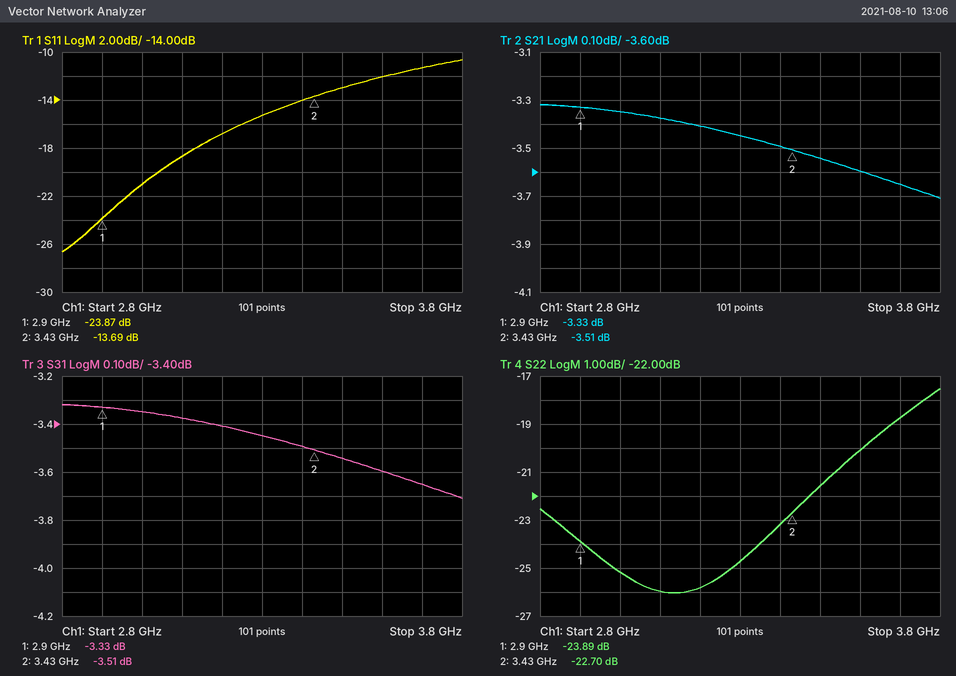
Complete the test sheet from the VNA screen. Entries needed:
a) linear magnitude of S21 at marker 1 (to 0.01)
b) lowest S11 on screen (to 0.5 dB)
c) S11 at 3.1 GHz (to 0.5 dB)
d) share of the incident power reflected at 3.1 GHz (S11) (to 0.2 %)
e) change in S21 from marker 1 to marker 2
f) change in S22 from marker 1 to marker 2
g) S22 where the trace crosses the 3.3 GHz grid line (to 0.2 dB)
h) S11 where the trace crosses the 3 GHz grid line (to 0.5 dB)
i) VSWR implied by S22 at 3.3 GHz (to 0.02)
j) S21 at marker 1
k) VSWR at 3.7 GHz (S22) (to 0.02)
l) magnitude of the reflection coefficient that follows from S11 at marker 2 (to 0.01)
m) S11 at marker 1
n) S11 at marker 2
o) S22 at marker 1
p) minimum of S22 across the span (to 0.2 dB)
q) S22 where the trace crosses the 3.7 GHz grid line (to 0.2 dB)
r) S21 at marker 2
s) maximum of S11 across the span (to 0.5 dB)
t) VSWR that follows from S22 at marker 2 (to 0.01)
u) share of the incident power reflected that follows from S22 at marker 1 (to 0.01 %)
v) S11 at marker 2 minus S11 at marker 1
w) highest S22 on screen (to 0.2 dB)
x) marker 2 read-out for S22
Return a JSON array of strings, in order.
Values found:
["0.68", "-26.5 dB", "-18.5 dB", "1.4 %", "-0.18 dB", "1.19 dB", "-24.8 dB", "-21.0 dB", "1.12", "-3.33 dB", "1.26", "0.21", "-23.87 dB", "-13.69 dB", "-23.89 dB", "-26.0 dB", "-18.8 dB", "-3.51 dB", "-10.5 dB", "1.16", "0.41 %", "10.18 dB", "-17.6 dB", "-22.70 dB"]
